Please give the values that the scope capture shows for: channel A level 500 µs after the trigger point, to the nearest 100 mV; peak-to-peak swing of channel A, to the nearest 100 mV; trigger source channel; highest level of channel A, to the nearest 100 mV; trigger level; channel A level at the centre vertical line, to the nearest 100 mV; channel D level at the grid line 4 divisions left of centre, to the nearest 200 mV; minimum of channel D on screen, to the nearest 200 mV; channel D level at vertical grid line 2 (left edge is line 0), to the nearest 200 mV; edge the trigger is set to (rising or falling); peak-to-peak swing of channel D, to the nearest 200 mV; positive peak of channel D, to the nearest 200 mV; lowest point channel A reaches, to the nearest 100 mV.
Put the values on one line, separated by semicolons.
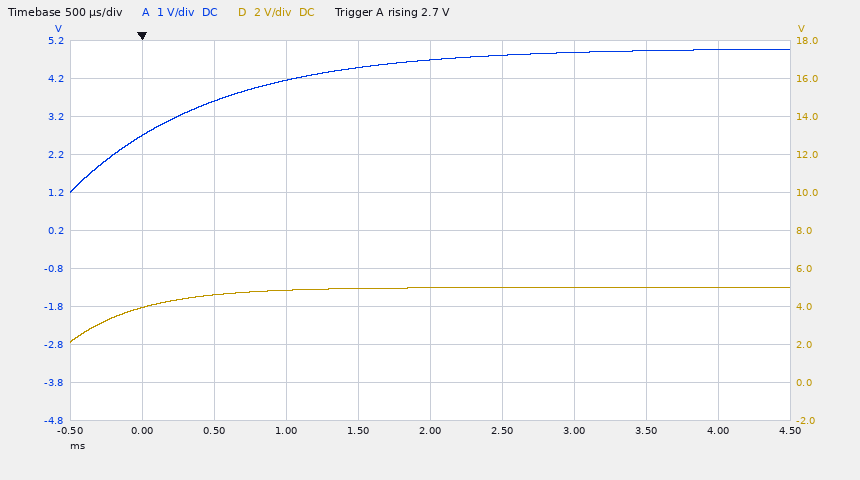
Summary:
3.6 V; 3.8 V; channel A; 5.0 V; 2.7 V; 4.7 V; 4.0 V; 2.2 V; 4.6 V; rising; 2.8 V; 5.0 V; 1.2 V
